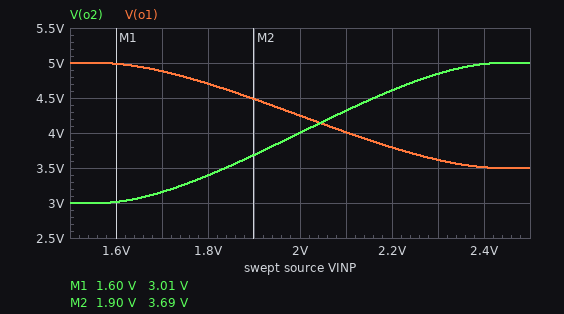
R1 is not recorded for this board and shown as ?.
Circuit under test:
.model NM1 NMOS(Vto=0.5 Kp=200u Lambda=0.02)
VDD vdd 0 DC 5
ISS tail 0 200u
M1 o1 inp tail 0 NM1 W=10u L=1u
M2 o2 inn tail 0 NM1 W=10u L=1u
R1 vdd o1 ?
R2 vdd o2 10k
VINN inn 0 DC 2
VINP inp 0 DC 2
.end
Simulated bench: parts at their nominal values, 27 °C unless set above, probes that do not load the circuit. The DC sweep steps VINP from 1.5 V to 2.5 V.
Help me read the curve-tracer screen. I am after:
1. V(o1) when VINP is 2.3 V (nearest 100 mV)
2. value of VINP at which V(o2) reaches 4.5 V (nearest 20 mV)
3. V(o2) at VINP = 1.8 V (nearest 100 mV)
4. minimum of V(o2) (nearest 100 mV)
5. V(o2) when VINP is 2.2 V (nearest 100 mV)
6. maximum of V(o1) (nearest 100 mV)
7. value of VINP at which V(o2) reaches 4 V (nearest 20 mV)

3.6 V
2.16 V
3.4 V
3.0 V
4.6 V
5.0 V
2.00 V
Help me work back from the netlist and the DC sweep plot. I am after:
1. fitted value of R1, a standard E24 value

7.5 kΩ
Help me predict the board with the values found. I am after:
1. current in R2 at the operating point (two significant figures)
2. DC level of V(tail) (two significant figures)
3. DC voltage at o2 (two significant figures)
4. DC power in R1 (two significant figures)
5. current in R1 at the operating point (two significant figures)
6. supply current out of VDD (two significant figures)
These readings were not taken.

100 µA
1.2 V
4.0 V
75 µW
100 µA
200 µA
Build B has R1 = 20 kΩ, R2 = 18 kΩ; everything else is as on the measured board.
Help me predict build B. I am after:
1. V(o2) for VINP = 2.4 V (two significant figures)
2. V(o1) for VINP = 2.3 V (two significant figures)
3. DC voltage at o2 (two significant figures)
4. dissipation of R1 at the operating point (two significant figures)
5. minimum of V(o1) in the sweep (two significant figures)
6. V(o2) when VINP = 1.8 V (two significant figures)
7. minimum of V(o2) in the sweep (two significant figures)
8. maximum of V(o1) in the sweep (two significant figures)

4.5 V
1.6 V
3.2 V
200 µW
1.5 V
2.1 V
1.4 V
5.0 V
